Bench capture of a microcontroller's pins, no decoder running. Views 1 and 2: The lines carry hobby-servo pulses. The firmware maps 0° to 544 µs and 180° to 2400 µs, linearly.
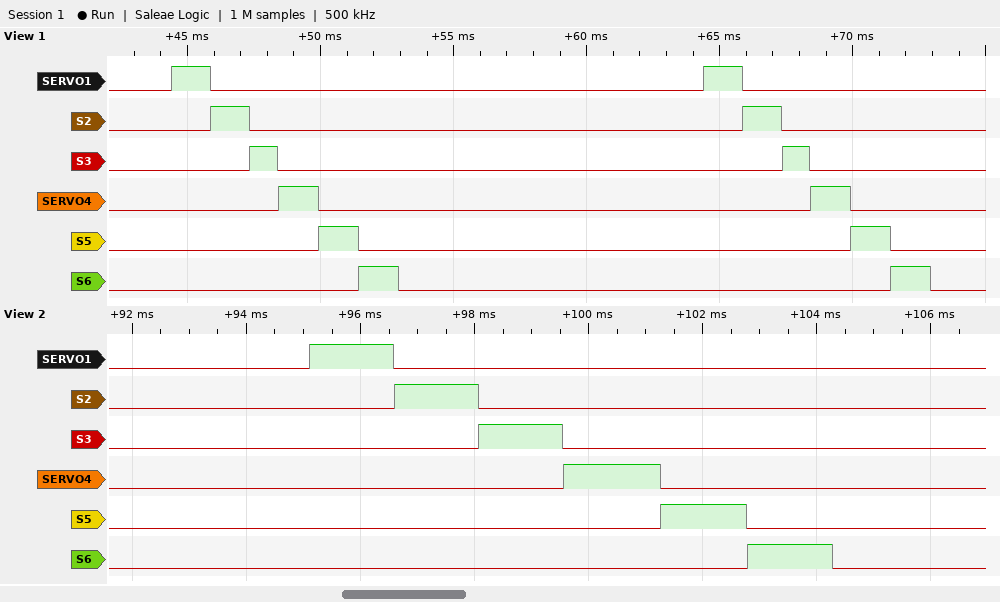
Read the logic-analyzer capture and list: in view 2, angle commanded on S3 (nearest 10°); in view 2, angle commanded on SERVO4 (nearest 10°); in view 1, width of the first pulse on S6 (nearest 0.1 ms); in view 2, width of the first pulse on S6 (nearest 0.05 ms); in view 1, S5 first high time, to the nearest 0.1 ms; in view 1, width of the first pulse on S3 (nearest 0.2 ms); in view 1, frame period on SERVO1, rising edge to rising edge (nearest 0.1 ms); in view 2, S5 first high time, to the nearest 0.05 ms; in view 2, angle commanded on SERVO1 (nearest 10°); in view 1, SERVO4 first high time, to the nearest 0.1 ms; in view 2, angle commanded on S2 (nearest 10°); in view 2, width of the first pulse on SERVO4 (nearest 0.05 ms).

90°
110°
1.5 ms
1.50 ms
1.5 ms
1.0 ms
20.0 ms
1.50 ms
90°
1.5 ms
90°
1.70 ms
